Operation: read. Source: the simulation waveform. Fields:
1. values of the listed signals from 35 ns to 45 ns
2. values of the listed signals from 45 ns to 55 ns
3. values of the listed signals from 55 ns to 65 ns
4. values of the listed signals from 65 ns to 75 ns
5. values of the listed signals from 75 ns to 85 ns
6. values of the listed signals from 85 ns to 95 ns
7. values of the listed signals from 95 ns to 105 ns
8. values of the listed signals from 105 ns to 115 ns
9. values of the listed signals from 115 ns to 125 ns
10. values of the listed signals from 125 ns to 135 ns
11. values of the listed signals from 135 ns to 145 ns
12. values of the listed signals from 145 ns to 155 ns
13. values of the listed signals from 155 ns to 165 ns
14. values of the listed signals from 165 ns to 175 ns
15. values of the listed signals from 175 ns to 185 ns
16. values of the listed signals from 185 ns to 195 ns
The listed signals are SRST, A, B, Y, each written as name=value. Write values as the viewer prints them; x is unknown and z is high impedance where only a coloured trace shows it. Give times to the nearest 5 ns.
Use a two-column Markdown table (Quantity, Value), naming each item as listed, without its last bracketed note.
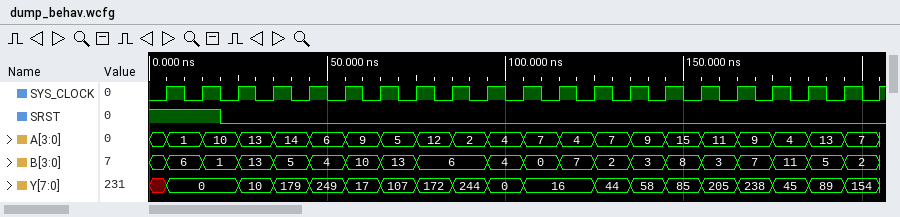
| Quantity | Value |
|---|---|
| values of the listed signals from 35 ns to 45 ns | SRST=0, A=14, B=5, Y=179 |
| values of the listed signals from 45 ns to 55 ns | SRST=0, A=6, B=4, Y=249 |
| values of the listed signals from 55 ns to 65 ns | SRST=0, A=9, B=10, Y=17 |
| values of the listed signals from 65 ns to 75 ns | SRST=0, A=5, B=13, Y=107 |
| values of the listed signals from 75 ns to 85 ns | SRST=0, A=12, B=6, Y=172 |
| values of the listed signals from 85 ns to 95 ns | SRST=0, A=2, B=6, Y=244 |
| values of the listed signals from 95 ns to 105 ns | SRST=0, A=4, B=4, Y=0 |
| values of the listed signals from 105 ns to 115 ns | SRST=0, A=7, B=0, Y=16 |
| values of the listed signals from 115 ns to 125 ns | SRST=0, A=4, B=7, Y=16 |
| values of the listed signals from 125 ns to 135 ns | SRST=0, A=7, B=2, Y=44 |
| values of the listed signals from 135 ns to 145 ns | SRST=0, A=9, B=3, Y=58 |
| values of the listed signals from 145 ns to 155 ns | SRST=0, A=15, B=8, Y=85 |
| values of the listed signals from 155 ns to 165 ns | SRST=0, A=11, B=3, Y=205 |
| values of the listed signals from 165 ns to 175 ns | SRST=0, A=9, B=7, Y=238 |
| values of the listed signals from 175 ns to 185 ns | SRST=0, A=4, B=11, Y=45 |
| values of the listed signals from 185 ns to 195 ns | SRST=0, A=13, B=5, Y=89 |
